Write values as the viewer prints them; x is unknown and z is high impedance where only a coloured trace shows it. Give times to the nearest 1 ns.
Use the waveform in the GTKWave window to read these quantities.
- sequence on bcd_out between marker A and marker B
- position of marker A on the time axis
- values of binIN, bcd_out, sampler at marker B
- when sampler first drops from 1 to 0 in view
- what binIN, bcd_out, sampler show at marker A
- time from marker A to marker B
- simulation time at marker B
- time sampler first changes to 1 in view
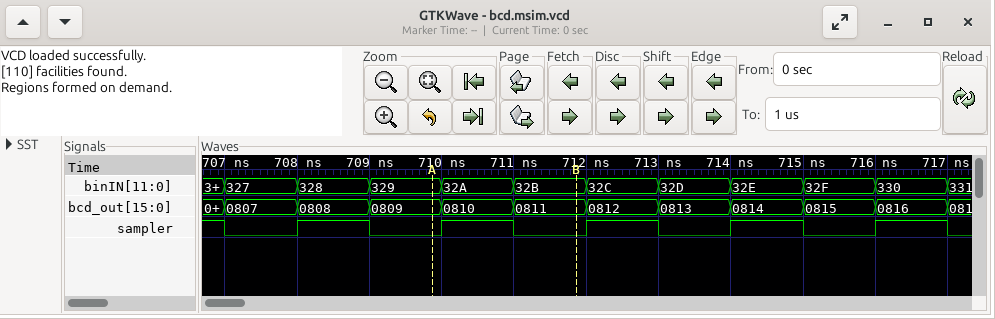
0809, 0810, 0811
710 ns
binIN=32B, bcd_out=0811, sampler=0
707 ns
binIN=329, bcd_out=0809, sampler=0
2 ns
712 ns
708 ns
